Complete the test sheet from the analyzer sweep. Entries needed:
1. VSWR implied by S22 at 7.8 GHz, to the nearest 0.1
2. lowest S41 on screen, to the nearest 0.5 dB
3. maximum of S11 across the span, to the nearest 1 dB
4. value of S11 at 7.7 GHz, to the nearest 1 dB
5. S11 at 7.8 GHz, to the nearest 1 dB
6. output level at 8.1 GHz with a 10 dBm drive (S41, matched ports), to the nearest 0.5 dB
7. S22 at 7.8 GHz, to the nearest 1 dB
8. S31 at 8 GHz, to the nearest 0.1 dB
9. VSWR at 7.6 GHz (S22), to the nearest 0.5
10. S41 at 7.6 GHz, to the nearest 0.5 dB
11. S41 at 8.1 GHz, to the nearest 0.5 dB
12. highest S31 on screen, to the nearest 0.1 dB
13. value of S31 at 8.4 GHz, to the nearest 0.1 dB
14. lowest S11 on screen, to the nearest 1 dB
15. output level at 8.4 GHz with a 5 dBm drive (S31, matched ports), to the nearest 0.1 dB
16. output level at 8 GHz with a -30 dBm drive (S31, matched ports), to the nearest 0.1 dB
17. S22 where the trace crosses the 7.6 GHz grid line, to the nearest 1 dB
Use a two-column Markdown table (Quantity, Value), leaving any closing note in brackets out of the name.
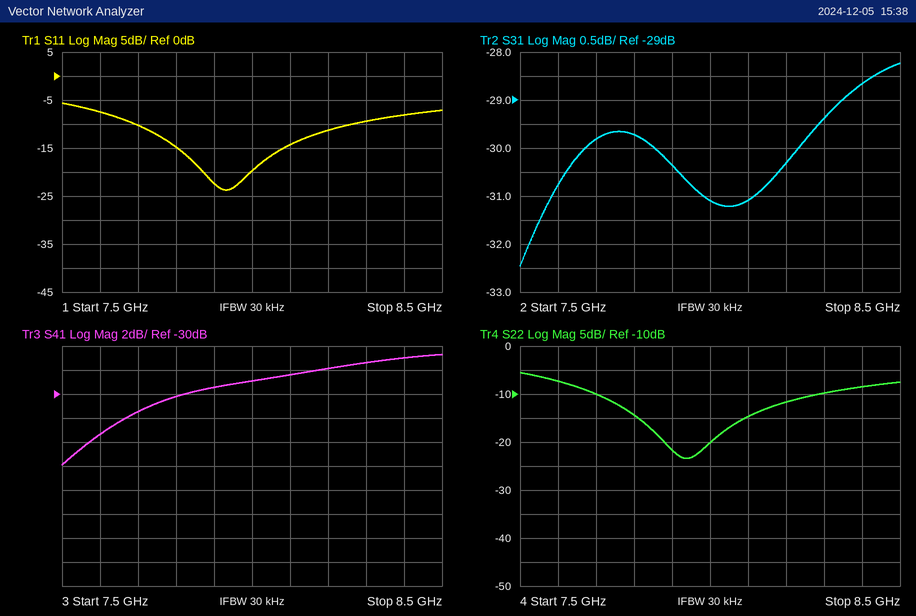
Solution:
| Quantity | Value |
|---|---|
| VSWR implied by S22 at 7.8 GHz, to the nearest 0.1 | 1.5 |
| lowest S41 on screen, to the nearest 0.5 dB | -36.0 dB |
| maximum of S11 across the span, to the nearest 1 dB | -6 dB |
| value of S11 at 7.7 GHz, to the nearest 1 dB | -10 dB |
| S11 at 7.8 GHz, to the nearest 1 dB | -15 dB |
| output level at 8.1 GHz with a 10 dBm drive (S41, matched ports), to the nearest 0.5 dB | -18.5 dBm |
| S22 at 7.8 GHz, to the nearest 1 dB | -14 dB |
| S31 at 8 GHz, to the nearest 0.1 dB | -31.1 dB |
| VSWR at 7.6 GHz (S22), to the nearest 0.5 | 2.5 |
| S41 at 7.6 GHz, to the nearest 0.5 dB | -33.5 dB |
| S41 at 8.1 GHz, to the nearest 0.5 dB | -28.5 dB |
| highest S31 on screen, to the nearest 0.1 dB | -28.2 dB |
| value of S31 at 8.4 GHz, to the nearest 0.1 dB | -28.7 dB |
| lowest S11 on screen, to the nearest 1 dB | -24 dB |
| output level at 8.4 GHz with a 5 dBm drive (S31, matched ports), to the nearest 0.1 dB | -23.7 dBm |
| output level at 8 GHz with a -30 dBm drive (S31, matched ports), to the nearest 0.1 dB | -61.1 dBm |
| S22 where the trace crosses the 7.6 GHz grid line, to the nearest 1 dB | -7 dB |
